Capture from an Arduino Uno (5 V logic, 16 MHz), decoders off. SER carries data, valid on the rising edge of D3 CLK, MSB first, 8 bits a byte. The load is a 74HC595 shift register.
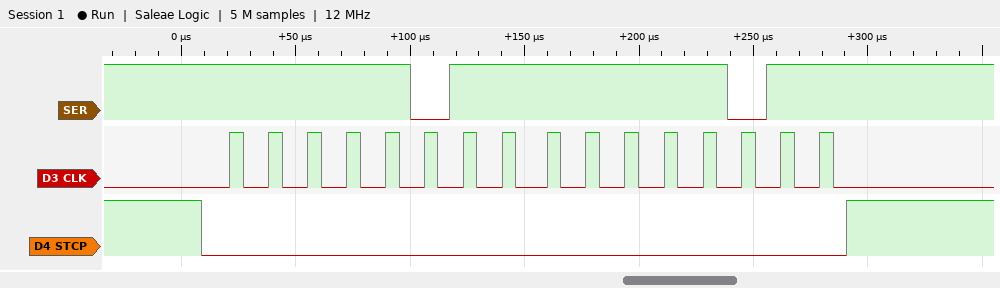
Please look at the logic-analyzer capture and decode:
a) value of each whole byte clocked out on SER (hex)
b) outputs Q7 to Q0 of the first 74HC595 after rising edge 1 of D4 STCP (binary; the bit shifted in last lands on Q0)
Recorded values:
0xFB 0xFB
11111011
